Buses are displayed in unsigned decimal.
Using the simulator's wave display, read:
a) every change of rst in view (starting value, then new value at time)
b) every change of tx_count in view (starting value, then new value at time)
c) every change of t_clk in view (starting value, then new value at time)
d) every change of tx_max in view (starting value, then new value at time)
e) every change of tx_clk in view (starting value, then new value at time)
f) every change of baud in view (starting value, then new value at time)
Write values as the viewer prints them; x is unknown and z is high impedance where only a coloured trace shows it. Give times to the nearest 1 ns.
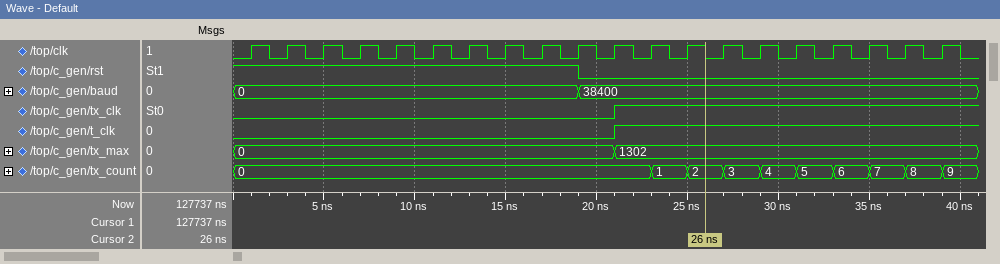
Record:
1, 0 at 19 ns
0, 1 at 23 ns, 2 at 25 ns, 3 at 27 ns, 4 at 29 ns, 5 at 31 ns, 6 at 33 ns, 7 at 35 ns, 8 at 37 ns, 9 at 39 ns
0, 1 at 21 ns
0, 1302 at 21 ns
0, 1 at 21 ns
0, 38400 at 19 ns
